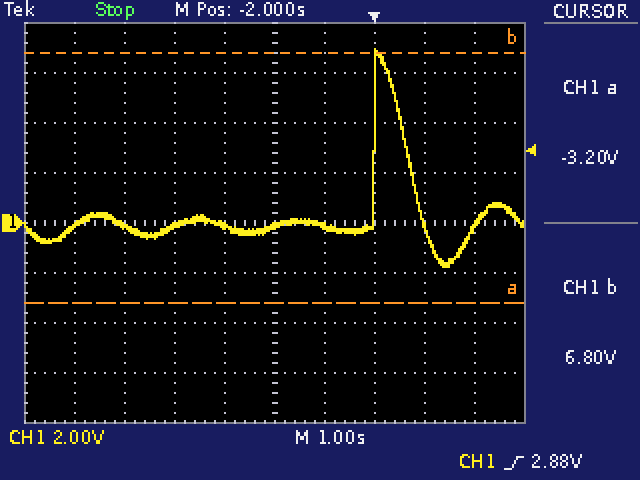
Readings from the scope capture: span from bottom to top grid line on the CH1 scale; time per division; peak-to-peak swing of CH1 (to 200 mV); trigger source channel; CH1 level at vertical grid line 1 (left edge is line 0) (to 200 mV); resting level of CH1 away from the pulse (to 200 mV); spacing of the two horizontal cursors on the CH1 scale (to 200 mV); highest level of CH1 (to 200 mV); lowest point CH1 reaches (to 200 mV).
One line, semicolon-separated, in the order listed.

16 V; 1 s; 8.8 V; CH1; -200 mV; -200 mV; 10.0 V; 7.0 V; -1.8 V
